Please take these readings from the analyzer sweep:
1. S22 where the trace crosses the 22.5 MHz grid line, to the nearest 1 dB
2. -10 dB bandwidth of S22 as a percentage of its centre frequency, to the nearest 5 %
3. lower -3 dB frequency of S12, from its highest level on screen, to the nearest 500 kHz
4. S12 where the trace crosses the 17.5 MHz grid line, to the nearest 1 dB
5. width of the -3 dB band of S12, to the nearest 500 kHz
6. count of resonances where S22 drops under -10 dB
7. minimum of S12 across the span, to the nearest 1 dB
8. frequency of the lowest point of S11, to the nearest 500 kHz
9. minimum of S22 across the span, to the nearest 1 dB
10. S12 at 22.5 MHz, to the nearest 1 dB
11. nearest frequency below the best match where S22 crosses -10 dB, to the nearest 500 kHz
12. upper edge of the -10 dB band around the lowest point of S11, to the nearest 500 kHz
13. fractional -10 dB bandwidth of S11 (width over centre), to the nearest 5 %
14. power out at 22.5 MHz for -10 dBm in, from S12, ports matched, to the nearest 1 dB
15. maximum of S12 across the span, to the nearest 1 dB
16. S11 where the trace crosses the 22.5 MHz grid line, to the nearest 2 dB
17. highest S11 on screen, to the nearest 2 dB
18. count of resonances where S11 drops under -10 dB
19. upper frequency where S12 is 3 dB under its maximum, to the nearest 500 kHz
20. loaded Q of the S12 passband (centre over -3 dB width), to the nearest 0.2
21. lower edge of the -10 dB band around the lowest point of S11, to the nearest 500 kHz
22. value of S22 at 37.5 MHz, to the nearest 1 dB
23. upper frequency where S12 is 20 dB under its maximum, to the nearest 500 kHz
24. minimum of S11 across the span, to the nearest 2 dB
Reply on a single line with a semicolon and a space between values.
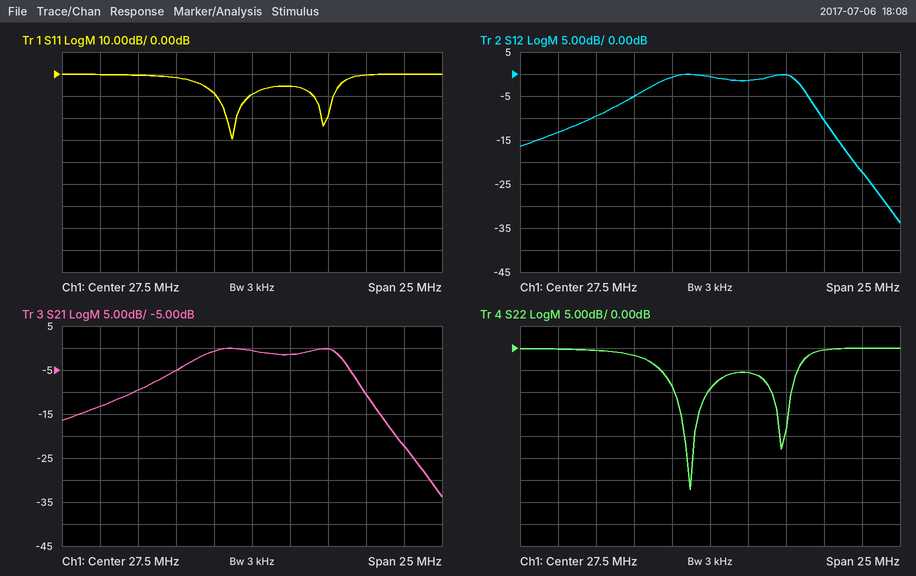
-2 dB; 10 %; 23.5 MHz; -13 dB; 10.0 MHz; 2; -34 dB; 26.0 MHz; -32 dB; -5 dB; 25.0 MHz; 27.5 MHz; 10 %; -15 dBm; 0 dB; -2 dB; 0 dB; 2; 33.5 MHz; 2.8; 25.0 MHz; 0 dB; 37.0 MHz; -30 dB
